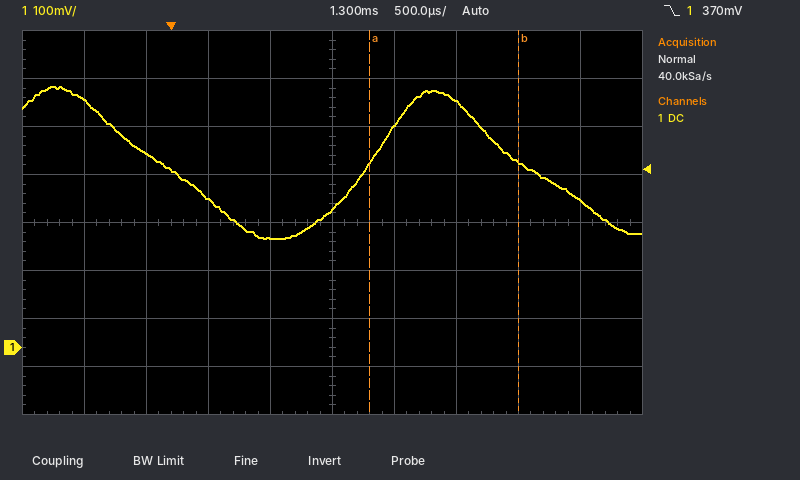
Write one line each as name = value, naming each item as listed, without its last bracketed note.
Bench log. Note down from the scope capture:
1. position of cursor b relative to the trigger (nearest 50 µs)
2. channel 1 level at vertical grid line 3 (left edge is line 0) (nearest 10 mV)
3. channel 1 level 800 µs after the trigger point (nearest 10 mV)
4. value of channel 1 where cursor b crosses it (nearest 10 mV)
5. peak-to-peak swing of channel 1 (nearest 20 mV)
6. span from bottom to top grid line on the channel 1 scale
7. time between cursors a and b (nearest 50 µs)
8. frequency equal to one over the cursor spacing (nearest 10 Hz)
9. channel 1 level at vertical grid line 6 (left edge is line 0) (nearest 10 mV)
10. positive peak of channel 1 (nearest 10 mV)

position of cursor b relative to the trigger = +2.80 ms
channel 1 level at vertical grid line 3 (left edge is line 0) = 310 mV
channel 1 level 800 µs after the trigger point = 230 mV
value of channel 1 where cursor b crosses it = 390 mV
peak-to-peak swing of channel 1 = 320 mV
span from bottom to top grid line on the channel 1 scale = 800 mV
time between cursors a and b = 1.20 ms
frequency equal to one over the cursor spacing = 830 Hz
channel 1 level at vertical grid line 6 (left edge is line 0) = 460 mV
positive peak of channel 1 = 540 mV
